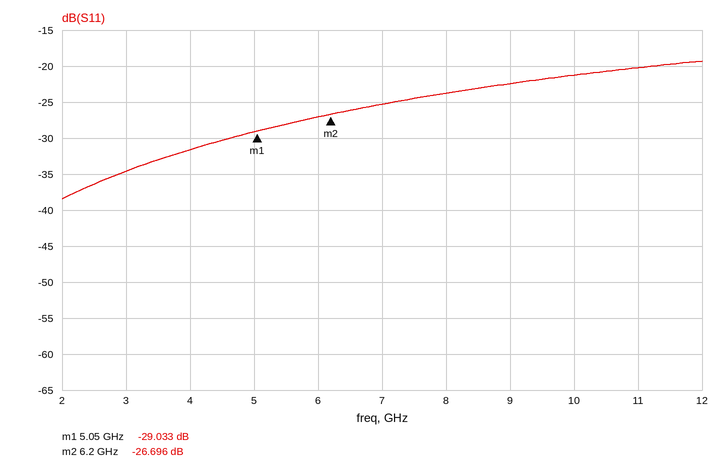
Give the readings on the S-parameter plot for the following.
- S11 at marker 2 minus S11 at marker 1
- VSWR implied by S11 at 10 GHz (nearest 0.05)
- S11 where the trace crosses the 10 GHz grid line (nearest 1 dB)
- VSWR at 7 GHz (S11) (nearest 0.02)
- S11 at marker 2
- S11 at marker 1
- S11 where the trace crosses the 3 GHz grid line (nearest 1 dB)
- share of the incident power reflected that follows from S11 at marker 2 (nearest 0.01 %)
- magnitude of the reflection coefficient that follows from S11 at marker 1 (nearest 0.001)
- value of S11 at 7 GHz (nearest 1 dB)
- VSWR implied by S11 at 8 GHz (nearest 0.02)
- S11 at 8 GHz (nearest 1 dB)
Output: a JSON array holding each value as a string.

["2.337 dB", "1.20", "-21 dB", "1.12", "-26.696 dB", "-29.033 dB", "-35 dB", "0.21 %", "0.035", "-25 dB", "1.14", "-24 dB"]
